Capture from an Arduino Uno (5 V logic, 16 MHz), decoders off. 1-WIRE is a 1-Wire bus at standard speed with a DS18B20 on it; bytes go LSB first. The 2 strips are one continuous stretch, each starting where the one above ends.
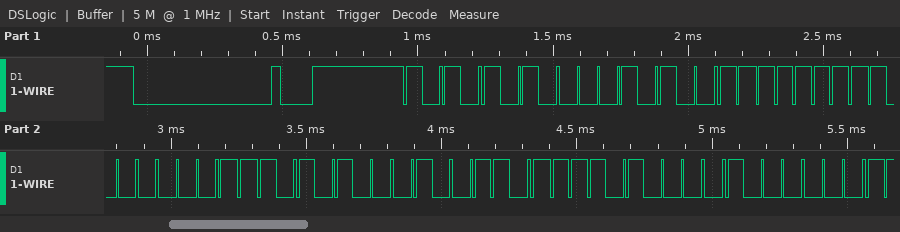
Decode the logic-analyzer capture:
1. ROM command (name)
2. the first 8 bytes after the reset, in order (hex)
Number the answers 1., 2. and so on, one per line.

1. Match ROM
2. 55 28 FF 81 2B B2 17 02
